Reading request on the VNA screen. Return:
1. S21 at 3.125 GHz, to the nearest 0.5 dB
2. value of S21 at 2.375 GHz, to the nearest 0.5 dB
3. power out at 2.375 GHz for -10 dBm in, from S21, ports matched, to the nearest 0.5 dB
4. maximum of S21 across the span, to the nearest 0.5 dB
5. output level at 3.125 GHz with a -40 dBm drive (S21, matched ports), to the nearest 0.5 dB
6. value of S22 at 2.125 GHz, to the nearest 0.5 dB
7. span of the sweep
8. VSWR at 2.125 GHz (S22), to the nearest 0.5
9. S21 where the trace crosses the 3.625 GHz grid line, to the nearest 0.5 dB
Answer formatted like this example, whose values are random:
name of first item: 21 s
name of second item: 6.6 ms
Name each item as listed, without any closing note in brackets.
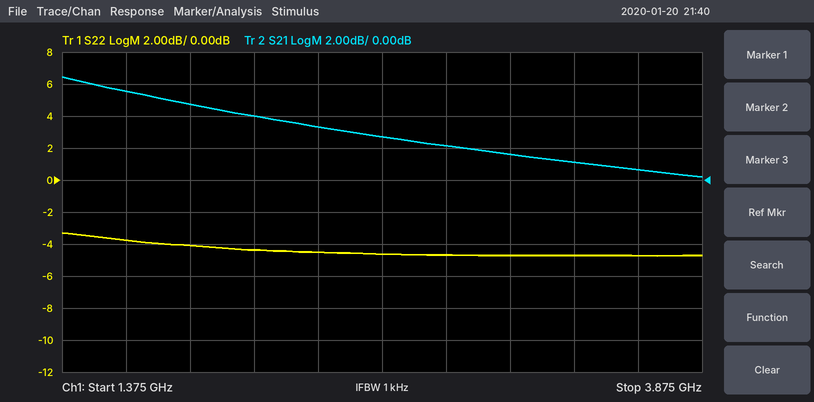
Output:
S21 at 3.125 GHz, to the nearest 0.5 dB: 1.5 dB
value of S21 at 2.375 GHz, to the nearest 0.5 dB: 3.5 dB
power out at 2.375 GHz for -10 dBm in, from S21, ports matched, to the nearest 0.5 dB: -6.5 dBm
maximum of S21 across the span, to the nearest 0.5 dB: 6.5 dB
output level at 3.125 GHz with a -40 dBm drive (S21, matched ports), to the nearest 0.5 dB: -38.5 dBm
value of S22 at 2.125 GHz, to the nearest 0.5 dB: -4.5 dB
span of the sweep: 2.5 GHz
VSWR at 2.125 GHz (S22), to the nearest 0.5: 4.0
S21 where the trace crosses the 3.625 GHz grid line, to the nearest 0.5 dB: 0.5 dB
